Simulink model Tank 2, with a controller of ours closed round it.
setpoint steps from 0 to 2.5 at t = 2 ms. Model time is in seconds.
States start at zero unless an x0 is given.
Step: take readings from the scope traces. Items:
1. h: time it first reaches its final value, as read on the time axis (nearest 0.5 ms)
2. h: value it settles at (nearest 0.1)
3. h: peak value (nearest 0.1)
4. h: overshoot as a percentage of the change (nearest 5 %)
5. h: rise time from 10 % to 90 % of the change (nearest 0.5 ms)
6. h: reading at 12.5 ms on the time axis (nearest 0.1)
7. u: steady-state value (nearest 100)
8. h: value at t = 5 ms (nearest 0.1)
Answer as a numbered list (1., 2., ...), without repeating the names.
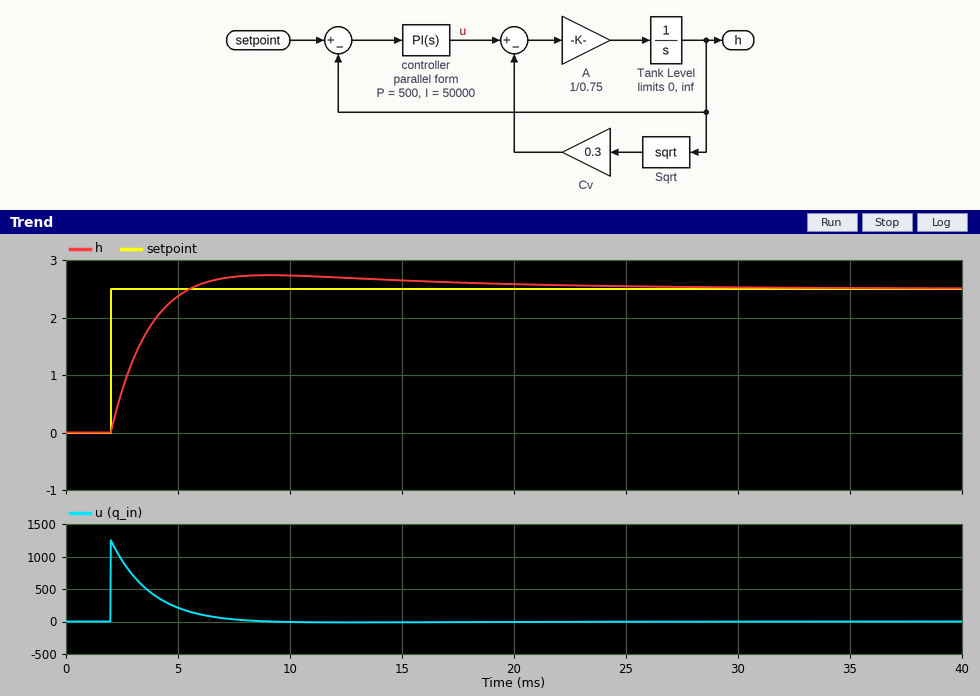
1. 5.5 ms
2. 2.5
3. 2.7
4. 10 %
5. 2.5 ms
6. 2.7
7. 0
8. 2.4
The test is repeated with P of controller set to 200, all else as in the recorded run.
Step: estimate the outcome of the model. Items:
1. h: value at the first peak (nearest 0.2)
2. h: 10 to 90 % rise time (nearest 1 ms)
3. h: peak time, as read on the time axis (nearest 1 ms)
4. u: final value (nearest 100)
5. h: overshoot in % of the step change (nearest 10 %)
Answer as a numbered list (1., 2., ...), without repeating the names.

1. 3.2
2. 4 ms
3. 11 ms
4. 0
5. 30 %
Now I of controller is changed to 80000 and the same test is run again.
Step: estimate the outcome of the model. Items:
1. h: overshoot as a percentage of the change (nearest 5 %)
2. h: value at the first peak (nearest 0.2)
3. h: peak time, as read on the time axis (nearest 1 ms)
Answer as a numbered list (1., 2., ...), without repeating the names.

1. 15 %
2. 2.8
3. 8 ms
